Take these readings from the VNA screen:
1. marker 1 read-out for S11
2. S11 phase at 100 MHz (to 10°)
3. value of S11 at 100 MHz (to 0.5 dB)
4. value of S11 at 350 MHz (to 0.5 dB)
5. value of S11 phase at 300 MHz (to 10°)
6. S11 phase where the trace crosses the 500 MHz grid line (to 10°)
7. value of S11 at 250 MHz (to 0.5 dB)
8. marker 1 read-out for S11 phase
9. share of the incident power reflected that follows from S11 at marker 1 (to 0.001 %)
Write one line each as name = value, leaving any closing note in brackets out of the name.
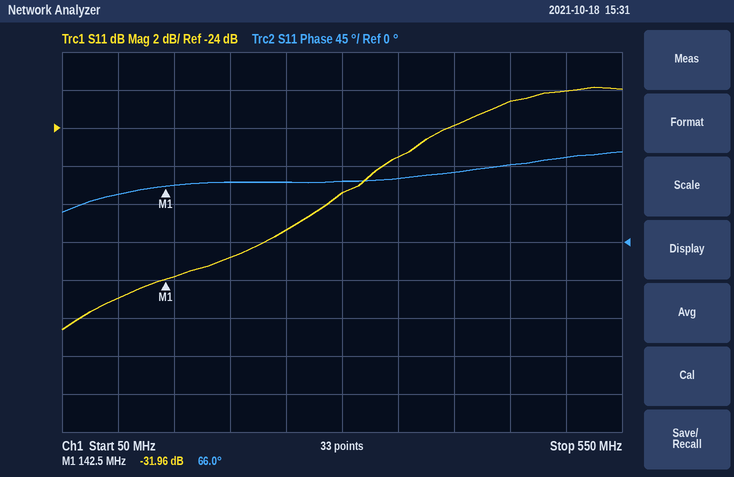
marker 1 read-out for S11 = -31.96 dB
S11 phase at 100 MHz = 60°
value of S11 at 100 MHz = -33.0 dB
value of S11 at 350 MHz = -25.5 dB
value of S11 phase at 300 MHz = 70°
S11 phase where the trace crosses the 500 MHz grid line = 100°
value of S11 at 250 MHz = -29.5 dB
marker 1 read-out for S11 phase = 66.0°
share of the incident power reflected that follows from S11 at marker 1 = 0.064 %
